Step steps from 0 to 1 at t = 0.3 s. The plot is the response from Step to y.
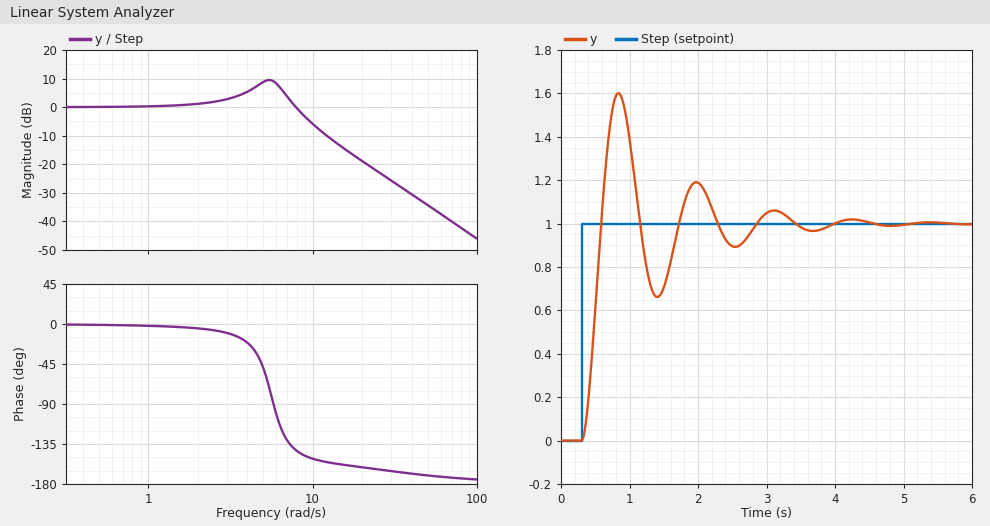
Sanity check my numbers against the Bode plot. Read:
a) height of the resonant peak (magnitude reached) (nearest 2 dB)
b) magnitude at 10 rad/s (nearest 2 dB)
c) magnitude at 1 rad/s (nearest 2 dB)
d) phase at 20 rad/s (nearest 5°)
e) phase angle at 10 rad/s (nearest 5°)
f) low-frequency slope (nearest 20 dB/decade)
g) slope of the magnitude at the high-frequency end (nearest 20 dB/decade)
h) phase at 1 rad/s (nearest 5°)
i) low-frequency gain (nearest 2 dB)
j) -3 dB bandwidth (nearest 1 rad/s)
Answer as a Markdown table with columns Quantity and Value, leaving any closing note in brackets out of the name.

| Quantity | Value |
|---|---|
| height of the resonant peak (magnitude reached) | 10 dB |
| magnitude at 10 rad/s | -6 dB |
| magnitude at 1 rad/s | 0 dB |
| phase at 20 rad/s | -160° |
| phase angle at 10 rad/s | -150° |
| low-frequency slope | 0 dB/decade |
| slope of the magnitude at the high-frequency end | -40 dB/decade |
| phase at 1 rad/s | 0° |
| low-frequency gain | 0 dB |
| -3 dB bandwidth | 9 rad/s |
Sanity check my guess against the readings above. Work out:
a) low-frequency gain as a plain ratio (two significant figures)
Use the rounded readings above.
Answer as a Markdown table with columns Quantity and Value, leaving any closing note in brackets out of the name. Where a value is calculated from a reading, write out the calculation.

| Quantity | Value |
|---|---|
| low-frequency gain as a plain ratio | 10^(0 / 20) = 1.0 |
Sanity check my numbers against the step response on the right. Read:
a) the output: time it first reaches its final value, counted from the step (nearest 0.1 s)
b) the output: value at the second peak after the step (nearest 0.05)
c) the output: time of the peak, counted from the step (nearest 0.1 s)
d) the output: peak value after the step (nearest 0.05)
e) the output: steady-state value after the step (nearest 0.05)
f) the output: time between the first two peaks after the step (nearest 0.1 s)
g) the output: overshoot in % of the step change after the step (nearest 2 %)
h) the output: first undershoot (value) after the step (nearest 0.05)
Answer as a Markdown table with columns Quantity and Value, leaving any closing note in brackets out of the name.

| Quantity | Value |
|---|---|
| the output: time it first reaches its final value, counted from the step | 0.3 s |
| the output: value at the second peak after the step | 1.20 |
| the output: time of the peak, counted from the step | 0.5 s |
| the output: peak value after the step | 1.60 |
| the output: steady-state value after the step | 1.00 |
| the output: time between the first two peaks after the step | 1.1 s |
| the output: overshoot in % of the step change after the step | 60 % |
| the output: first undershoot (value) after the step | 0.65 |
